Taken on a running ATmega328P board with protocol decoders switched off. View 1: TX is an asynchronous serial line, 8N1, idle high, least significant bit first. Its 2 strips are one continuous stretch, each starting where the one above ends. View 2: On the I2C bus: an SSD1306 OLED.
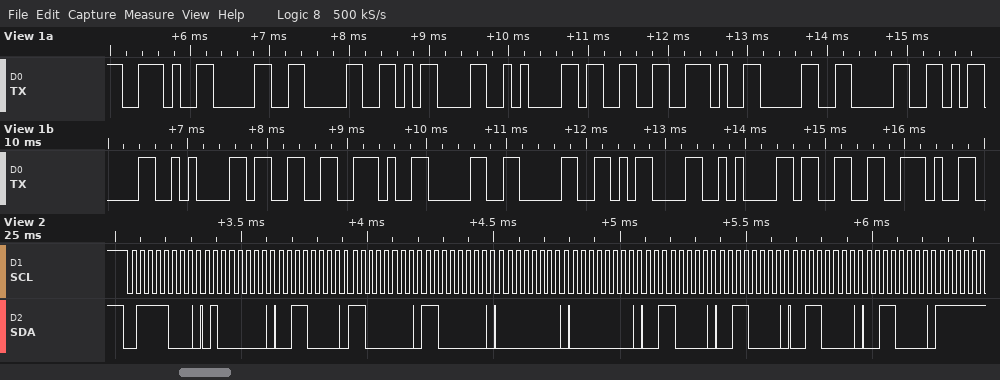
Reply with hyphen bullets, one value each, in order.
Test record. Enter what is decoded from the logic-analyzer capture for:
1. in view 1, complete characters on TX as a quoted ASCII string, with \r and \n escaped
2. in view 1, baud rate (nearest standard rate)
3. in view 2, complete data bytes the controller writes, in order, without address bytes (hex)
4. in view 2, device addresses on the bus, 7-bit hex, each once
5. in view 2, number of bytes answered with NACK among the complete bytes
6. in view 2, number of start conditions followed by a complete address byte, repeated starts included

- ".00\r\n3.00\r\n3.00\r\n3."
- 9600 baud
- 40 30 C0 C0 00 00 30 30 30 30
- 0x3C
- 0
- 1
